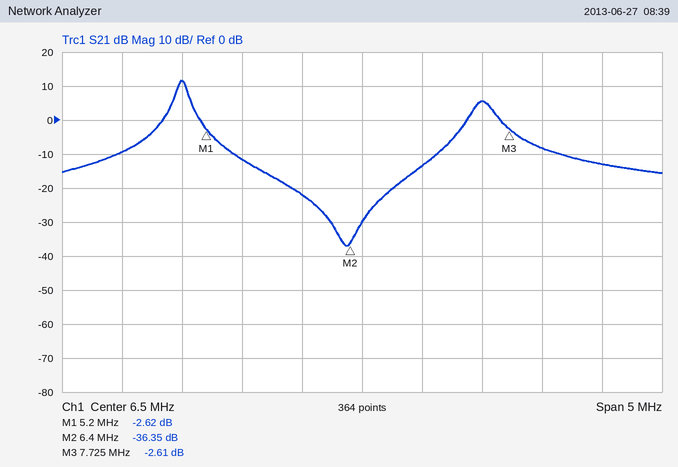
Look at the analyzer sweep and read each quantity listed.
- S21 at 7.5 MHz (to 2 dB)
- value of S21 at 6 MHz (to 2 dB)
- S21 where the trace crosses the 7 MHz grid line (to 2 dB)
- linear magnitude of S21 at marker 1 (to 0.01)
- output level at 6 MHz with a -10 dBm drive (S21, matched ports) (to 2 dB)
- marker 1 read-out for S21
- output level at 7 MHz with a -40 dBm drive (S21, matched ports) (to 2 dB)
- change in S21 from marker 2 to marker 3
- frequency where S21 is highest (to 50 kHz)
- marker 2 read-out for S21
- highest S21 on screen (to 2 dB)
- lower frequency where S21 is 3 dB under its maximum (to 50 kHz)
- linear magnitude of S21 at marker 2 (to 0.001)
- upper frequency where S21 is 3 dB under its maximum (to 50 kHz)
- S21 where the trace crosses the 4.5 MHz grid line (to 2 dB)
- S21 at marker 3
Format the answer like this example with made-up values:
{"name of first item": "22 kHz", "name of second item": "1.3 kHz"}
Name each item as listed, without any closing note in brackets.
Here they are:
{"S21 at 7.5 MHz": "6 dB", "value of S21 at 6 MHz": "-22 dB", "S21 where the trace crosses the 7 MHz grid line": "-14 dB", "linear magnitude of S21 at marker 1": "0.74", "output level at 6 MHz with a -10 dBm drive (S21, matched ports)": "-32 dBm", "marker 1 read-out for S21": "-2.62 dB", "output level at 7 MHz with a -40 dBm drive (S21, matched ports)": "-54 dBm", "change in S21 from marker 2 to marker 3": "33.74 dB", "frequency where S21 is highest": "5.00 MHz", "marker 2 read-out for S21": "-36.35 dB", "highest S21 on screen": "12 dB", "lower frequency where S21 is 3 dB under its maximum": "4.95 MHz", "linear magnitude of S21 at marker 2": "0.015", "upper frequency where S21 is 3 dB under its maximum": "5.05 MHz", "S21 where the trace crosses the 4.5 MHz grid line": "-10 dB", "S21 at marker 3": "-2.61 dB"}
